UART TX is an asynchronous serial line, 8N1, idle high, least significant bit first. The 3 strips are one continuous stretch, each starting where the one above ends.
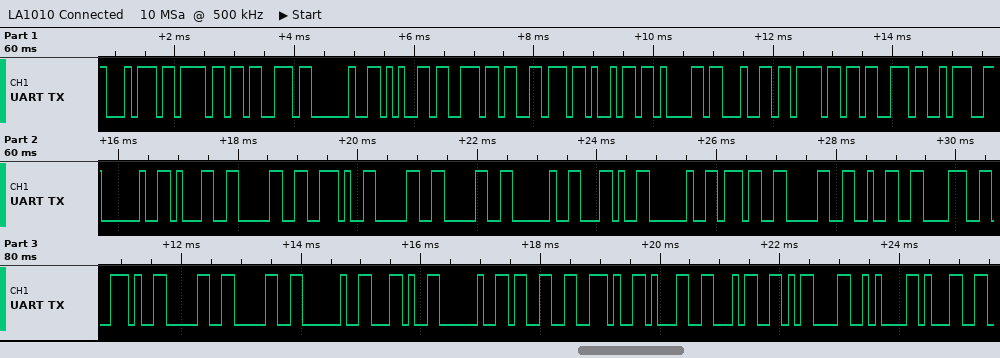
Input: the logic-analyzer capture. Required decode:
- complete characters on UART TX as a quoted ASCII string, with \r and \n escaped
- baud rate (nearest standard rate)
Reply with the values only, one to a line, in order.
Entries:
"tos enviados: 10.00 , 7028.00 , 3.14\r\n1"
9600 baud
